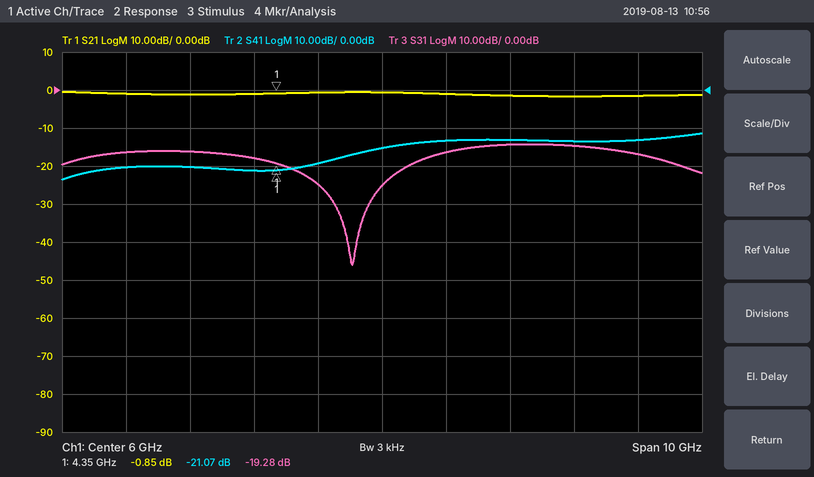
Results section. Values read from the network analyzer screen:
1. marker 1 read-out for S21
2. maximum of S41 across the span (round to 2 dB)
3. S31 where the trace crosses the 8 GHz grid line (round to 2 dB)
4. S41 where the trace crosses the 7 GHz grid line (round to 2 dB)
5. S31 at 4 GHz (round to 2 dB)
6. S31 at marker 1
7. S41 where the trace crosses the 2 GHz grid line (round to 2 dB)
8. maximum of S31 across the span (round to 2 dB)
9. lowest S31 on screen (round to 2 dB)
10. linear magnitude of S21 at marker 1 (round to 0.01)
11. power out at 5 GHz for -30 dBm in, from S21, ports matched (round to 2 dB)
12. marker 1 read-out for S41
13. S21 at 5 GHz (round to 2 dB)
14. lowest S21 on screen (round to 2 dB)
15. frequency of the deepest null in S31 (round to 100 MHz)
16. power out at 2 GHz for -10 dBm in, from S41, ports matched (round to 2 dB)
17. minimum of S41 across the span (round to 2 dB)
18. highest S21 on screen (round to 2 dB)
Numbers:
-0.85 dB
-12 dB
-14 dB
-14 dB
-18 dB
-19.28 dB
-20 dB
-14 dB
-46 dB
0.91
-30 dBm
-21.07 dB
0 dB
-2 dB
5.5 GHz
-30 dBm
-24 dB
0 dB
